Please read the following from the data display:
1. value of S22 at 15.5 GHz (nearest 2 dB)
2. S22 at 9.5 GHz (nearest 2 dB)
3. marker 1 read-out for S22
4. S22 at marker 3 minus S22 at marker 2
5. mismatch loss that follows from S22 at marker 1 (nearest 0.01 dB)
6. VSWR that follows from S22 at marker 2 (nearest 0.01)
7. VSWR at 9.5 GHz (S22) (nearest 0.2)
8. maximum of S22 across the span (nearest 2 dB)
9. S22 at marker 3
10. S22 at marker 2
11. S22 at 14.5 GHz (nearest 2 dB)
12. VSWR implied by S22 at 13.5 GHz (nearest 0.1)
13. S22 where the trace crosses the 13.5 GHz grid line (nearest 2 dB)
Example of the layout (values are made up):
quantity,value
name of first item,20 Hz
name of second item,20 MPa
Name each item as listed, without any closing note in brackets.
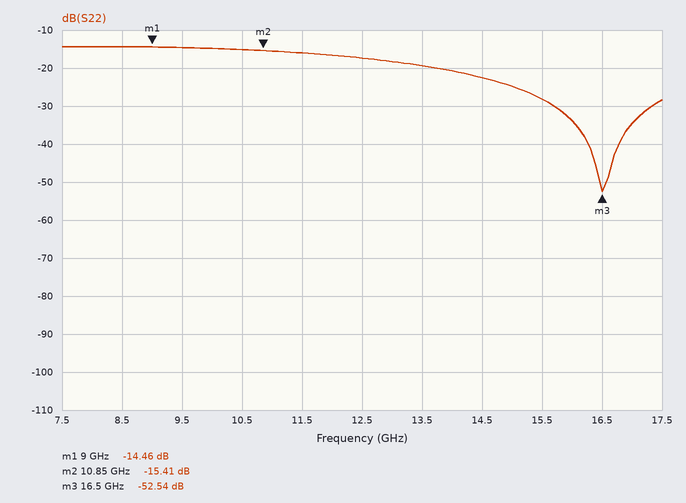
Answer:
quantity,value
value of S22 at 15.5 GHz,-28 dB
S22 at 9.5 GHz,-14 dB
marker 1 read-out for S22,-14.46 dB
S22 at marker 3 minus S22 at marker 2,-37.13 dB
mismatch loss that follows from S22 at marker 1,0.16 dB
VSWR that follows from S22 at marker 2,1.41
VSWR at 9.5 GHz (S22),1.4
maximum of S22 across the span,-14 dB
S22 at marker 3,-52.54 dB
S22 at marker 2,-15.41 dB
S22 at 14.5 GHz,-22 dB
VSWR implied by S22 at 13.5 GHz,1.2
S22 where the trace crosses the 13.5 GHz grid line,-20 dB
